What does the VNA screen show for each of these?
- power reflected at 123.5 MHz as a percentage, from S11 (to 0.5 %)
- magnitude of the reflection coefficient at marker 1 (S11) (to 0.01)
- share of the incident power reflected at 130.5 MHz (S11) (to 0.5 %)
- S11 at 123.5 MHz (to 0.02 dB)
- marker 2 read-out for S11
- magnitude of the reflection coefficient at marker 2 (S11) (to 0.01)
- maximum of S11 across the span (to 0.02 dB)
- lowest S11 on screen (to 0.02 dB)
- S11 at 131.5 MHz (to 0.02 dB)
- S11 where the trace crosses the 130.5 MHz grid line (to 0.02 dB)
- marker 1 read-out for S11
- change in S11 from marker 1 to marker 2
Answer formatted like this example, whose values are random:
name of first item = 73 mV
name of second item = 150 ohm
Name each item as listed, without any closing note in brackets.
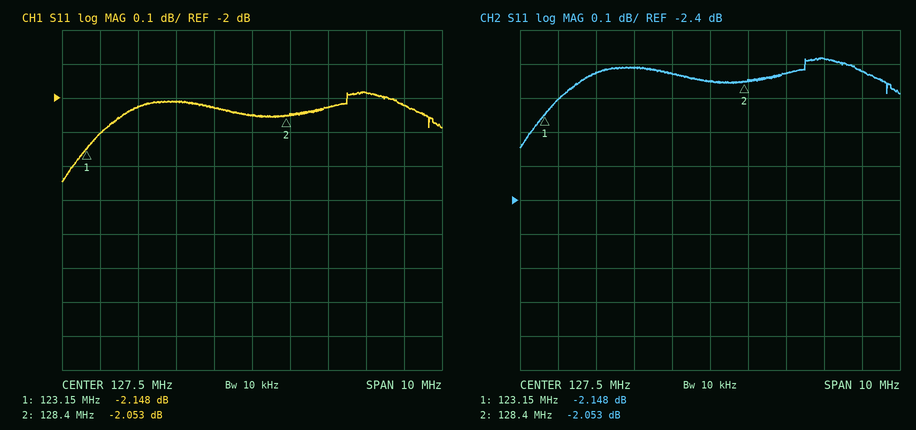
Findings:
power reflected at 123.5 MHz as a percentage, from S11 = 61.5 %
magnitude of the reflection coefficient at marker 1 (S11) = 0.78
share of the incident power reflected at 130.5 MHz (S11) = 63.5 %
S11 at 123.5 MHz = -2.10 dB
marker 2 read-out for S11 = -2.053 dB
magnitude of the reflection coefficient at marker 2 (S11) = 0.79
maximum of S11 across the span = -1.98 dB
lowest S11 on screen = -2.24 dB
S11 at 131.5 MHz = -2.02 dB
S11 where the trace crosses the 130.5 MHz grid line = -1.98 dB
marker 1 read-out for S11 = -2.148 dB
change in S11 from marker 1 to marker 2 = 0.095 dB
